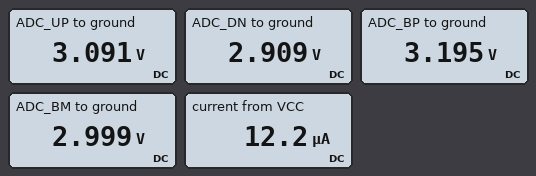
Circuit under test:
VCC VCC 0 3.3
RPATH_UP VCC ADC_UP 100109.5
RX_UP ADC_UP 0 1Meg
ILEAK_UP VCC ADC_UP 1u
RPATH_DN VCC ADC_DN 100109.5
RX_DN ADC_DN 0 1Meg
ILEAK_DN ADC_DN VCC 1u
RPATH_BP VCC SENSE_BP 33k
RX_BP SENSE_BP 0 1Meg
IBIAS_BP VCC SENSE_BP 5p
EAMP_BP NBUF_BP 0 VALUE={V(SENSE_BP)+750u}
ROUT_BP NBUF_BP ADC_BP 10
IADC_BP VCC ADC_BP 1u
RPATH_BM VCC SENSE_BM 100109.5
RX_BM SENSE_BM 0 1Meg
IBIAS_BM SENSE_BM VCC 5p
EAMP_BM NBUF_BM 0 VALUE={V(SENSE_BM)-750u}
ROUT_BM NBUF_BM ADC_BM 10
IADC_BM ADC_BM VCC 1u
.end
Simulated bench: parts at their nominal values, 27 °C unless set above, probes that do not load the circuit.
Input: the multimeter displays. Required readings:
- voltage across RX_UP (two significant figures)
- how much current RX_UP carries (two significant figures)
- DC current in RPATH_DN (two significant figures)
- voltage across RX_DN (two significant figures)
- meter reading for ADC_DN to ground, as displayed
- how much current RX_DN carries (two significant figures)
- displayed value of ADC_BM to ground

3.1 V
3.1 µA
3.9 µA
2.9 V
2.909 V
2.9 µA
2.999 V
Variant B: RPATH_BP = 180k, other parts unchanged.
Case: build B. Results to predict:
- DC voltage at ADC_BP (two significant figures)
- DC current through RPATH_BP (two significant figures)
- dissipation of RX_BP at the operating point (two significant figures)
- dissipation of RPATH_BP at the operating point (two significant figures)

2.8 V
2.8 µA
7.8 µW
1.4 µW
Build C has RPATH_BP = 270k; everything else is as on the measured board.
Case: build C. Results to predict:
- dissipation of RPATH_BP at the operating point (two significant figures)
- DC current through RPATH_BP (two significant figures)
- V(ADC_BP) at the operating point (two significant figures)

1.8 µW
2.6 µA
2.6 V
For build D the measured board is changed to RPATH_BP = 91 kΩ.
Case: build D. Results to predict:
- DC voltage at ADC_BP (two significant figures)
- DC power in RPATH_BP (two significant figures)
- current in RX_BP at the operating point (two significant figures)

3.0 V
830 nW
3.0 µA
